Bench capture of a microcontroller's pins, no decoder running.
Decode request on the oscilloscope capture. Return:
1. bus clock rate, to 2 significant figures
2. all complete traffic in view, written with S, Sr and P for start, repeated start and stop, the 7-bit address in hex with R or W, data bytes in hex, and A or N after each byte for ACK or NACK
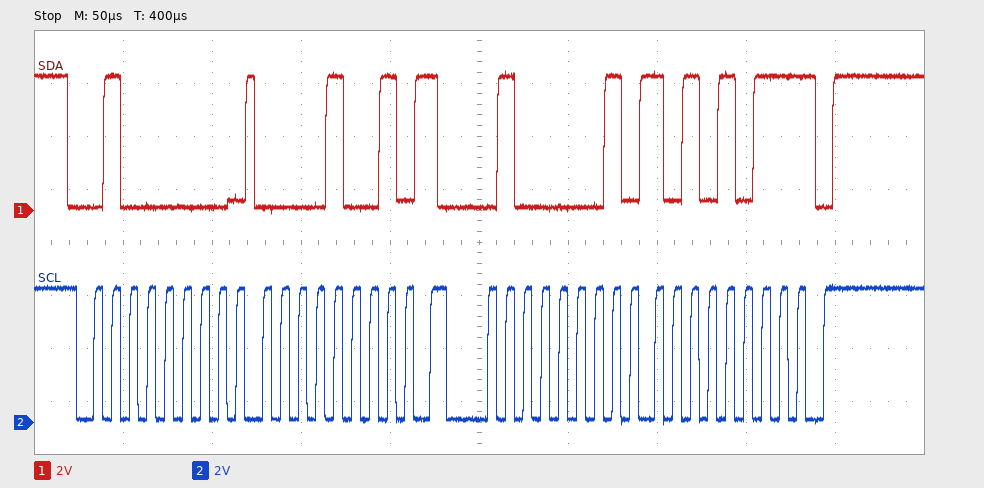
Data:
100 kHz
S 20W A 09 A Sr 20R A AB N P
